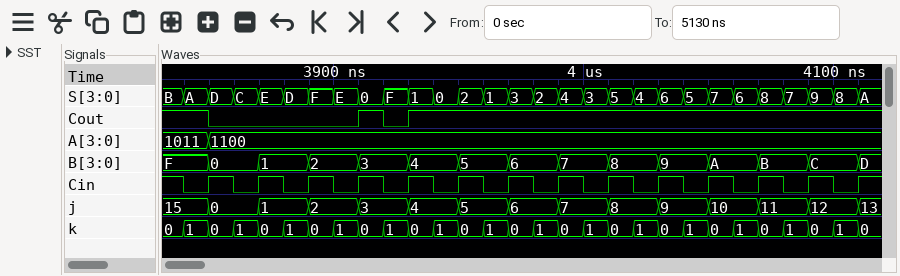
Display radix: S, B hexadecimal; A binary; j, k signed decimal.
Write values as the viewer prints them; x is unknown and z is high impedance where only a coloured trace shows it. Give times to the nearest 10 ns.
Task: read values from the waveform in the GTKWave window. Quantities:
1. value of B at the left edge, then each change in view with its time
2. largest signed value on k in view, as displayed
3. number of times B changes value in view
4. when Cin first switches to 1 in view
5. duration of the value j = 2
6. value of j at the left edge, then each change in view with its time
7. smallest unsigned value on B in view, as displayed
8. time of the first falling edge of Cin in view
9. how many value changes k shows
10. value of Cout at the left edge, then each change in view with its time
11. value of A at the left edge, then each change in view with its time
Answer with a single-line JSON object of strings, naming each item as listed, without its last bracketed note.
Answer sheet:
{"value of B at the left edge, then each change in view with its time": "F, 0 at 3850 ns, 1 at 3870 ns, 2 at 3890 ns, 3 at 3910 ns, 4 at 3930 ns, 5 at 3950 ns, 6 at 3970 ns, 7 at 3990 ns, 8 at 4010 ns, 9 at 4030 ns, A at 4050 ns, B at 4070 ns, C at 4090 ns, D at 4110 ns", "largest signed value on k in view, as displayed": "1", "number of times B changes value in view": "14", "when Cin first switches to 1 in view": "3850 ns", "duration of the value j = 2": "20 ns", "value of j at the left edge, then each change in view with its time": "15, 0 at 3850 ns, 1 at 3870 ns, 2 at 3890 ns, 3 at 3910 ns, 4 at 3930 ns, 5 at 3950 ns, 6 at 3970 ns, 7 at 3990 ns, 8 at 4010 ns, 9 at 4030 ns, 10 at 4050 ns, 11 at 4070 ns, 12 at 4090 ns, 13 at 4110 ns", "smallest unsigned value on B in view, as displayed": "0", "time of the first falling edge of Cin in view": "3840 ns", "how many value changes k shows": "28", "value of Cout at the left edge, then each change in view with its time": "1, 0 at 3850 ns, 1 at 3910 ns, 0 at 3920 ns, 1 at 3930 ns", "value of A at the left edge, then each change in view with its time": "1011, 1100 at 3850 ns"}
